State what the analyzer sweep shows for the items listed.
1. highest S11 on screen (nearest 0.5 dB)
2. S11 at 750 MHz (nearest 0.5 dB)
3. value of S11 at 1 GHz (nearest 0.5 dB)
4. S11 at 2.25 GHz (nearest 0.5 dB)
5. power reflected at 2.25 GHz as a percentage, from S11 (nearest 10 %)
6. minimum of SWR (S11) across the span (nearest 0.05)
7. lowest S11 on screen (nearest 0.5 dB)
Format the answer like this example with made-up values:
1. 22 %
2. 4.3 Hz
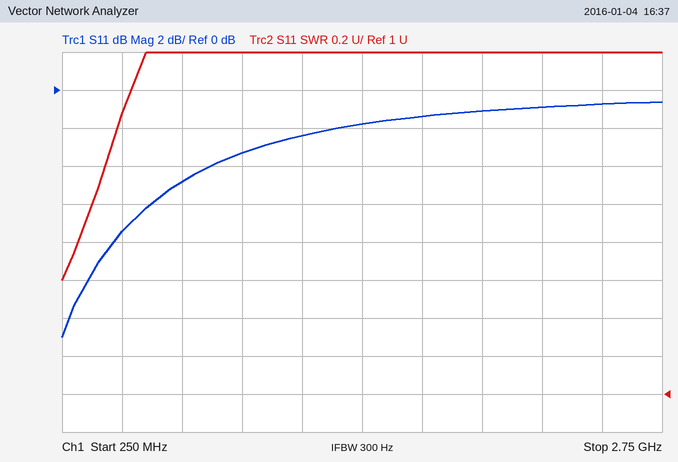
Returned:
1. -0.5 dB
2. -5.0 dB
3. -3.5 dB
4. -1.0 dB
5. 80 %
6. 1.60
7. -13.0 dB
